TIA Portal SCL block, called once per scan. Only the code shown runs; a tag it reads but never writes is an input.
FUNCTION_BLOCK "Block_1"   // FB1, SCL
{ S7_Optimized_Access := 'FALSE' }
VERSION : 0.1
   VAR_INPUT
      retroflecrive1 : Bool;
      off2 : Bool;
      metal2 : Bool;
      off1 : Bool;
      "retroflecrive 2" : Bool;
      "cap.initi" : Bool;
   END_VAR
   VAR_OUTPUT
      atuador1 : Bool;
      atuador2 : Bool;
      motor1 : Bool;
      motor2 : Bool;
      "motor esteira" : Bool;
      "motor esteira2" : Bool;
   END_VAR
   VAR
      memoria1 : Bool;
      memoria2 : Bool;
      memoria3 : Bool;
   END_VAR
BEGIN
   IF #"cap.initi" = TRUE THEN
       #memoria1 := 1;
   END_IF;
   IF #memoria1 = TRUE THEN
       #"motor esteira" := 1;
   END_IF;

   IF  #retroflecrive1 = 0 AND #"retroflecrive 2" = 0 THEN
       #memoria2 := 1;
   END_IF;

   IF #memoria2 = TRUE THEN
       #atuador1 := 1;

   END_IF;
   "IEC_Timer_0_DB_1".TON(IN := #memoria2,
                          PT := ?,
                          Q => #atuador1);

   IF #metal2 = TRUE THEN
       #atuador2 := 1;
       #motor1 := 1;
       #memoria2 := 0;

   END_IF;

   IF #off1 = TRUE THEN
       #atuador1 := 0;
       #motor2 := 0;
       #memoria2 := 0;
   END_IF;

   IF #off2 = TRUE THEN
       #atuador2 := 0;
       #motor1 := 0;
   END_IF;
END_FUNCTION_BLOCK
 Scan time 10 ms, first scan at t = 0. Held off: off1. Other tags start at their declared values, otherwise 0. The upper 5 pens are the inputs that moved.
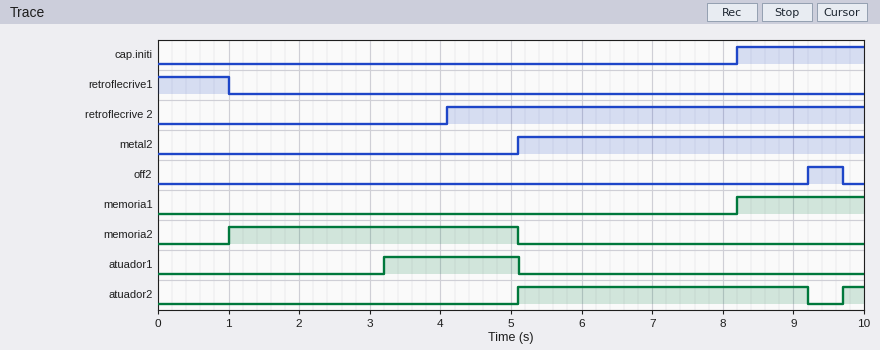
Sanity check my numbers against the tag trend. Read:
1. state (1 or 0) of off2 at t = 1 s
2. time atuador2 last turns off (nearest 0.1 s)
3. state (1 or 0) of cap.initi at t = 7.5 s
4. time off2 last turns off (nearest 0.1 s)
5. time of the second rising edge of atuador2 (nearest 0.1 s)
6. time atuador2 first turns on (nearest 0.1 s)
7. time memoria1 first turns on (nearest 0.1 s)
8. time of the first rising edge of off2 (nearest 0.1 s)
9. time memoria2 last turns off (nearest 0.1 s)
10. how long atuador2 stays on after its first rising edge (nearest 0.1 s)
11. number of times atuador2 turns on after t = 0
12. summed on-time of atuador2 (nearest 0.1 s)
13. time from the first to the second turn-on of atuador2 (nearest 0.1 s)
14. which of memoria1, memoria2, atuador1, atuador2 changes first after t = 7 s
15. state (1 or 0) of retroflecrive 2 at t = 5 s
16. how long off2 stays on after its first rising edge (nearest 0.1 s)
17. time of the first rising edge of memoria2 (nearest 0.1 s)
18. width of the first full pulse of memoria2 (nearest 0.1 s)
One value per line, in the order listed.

0
9.2 s
0
9.7 s
9.7 s
5.1 s
8.2 s
9.2 s
5.1 s
4.1 s
2
4.4 s
4.6 s
memoria1
1
0.5 s
1.0 s
4.1 s
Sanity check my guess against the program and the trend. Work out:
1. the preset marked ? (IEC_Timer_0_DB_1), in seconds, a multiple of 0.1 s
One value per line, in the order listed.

2.2 s
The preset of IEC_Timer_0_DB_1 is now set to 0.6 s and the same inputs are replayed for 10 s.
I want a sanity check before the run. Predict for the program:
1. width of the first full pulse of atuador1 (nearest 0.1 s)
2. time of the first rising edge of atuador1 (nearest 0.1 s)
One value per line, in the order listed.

3.5 s
1.6 s
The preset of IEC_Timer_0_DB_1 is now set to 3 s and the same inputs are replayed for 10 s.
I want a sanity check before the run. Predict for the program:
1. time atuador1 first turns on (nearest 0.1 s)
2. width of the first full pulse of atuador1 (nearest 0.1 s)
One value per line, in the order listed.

4.0 s
1.1 s
